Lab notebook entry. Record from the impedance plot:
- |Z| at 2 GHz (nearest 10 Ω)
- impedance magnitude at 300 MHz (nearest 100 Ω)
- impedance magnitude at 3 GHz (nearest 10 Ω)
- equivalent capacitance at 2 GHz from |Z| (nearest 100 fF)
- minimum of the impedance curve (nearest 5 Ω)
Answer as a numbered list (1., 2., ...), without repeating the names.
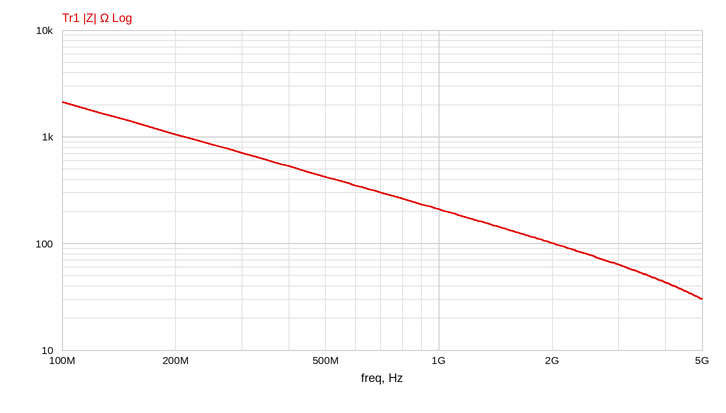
1. 100 Ω
2. 700 Ω
3. 60 Ω
4. 800 fF
5. 30 Ω
